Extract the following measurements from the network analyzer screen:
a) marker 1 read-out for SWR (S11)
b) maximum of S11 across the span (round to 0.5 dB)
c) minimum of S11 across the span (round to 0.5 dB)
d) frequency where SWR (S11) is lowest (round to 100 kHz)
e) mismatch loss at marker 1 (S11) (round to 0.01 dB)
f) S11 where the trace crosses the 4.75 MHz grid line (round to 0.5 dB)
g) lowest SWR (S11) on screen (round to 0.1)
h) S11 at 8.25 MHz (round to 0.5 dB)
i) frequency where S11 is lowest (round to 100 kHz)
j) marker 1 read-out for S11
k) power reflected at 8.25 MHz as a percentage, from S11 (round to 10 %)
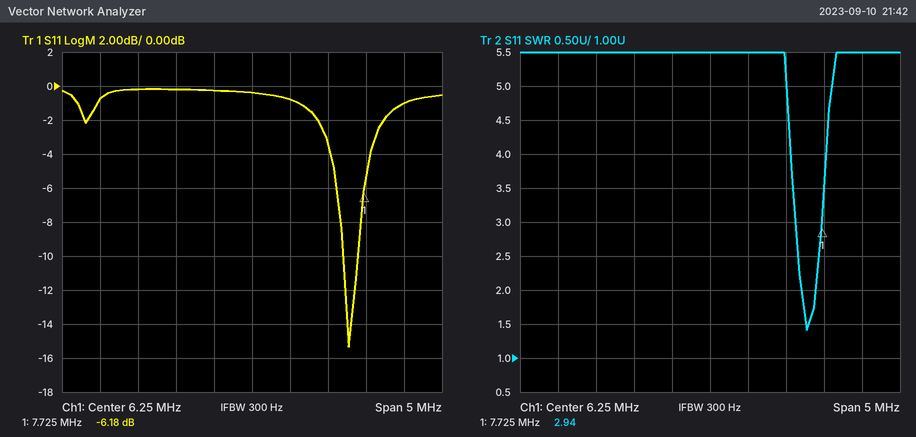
2.94
0.0 dB
-15.5 dB
7.5 MHz
1.20 dB
0.0 dB
1.4
-1.0 dB
7.5 MHz
-6.18 dB
80 %
